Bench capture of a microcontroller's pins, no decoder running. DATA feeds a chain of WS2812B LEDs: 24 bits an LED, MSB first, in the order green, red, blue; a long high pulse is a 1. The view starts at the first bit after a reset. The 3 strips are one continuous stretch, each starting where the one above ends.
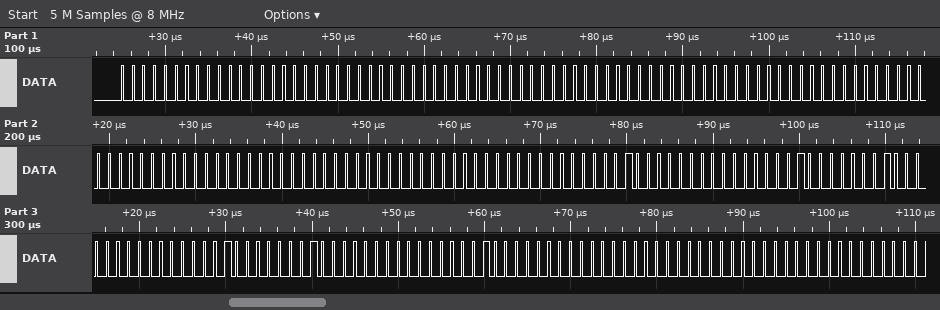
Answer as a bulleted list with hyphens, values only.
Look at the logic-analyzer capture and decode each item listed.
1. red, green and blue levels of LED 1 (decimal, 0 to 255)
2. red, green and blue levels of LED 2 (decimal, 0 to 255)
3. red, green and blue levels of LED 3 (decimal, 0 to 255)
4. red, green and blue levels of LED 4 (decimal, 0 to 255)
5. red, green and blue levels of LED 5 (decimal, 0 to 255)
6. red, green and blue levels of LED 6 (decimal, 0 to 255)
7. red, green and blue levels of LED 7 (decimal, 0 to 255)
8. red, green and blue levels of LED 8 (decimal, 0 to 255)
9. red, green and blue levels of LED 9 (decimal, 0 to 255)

- 0, 0, 0
- 0, 0, 0
- 0, 0, 0
- 0, 0, 0
- 0, 0, 0
- 0, 8, 8
- 0, 8, 8
- 0, 8, 8
- 0, 0, 0
